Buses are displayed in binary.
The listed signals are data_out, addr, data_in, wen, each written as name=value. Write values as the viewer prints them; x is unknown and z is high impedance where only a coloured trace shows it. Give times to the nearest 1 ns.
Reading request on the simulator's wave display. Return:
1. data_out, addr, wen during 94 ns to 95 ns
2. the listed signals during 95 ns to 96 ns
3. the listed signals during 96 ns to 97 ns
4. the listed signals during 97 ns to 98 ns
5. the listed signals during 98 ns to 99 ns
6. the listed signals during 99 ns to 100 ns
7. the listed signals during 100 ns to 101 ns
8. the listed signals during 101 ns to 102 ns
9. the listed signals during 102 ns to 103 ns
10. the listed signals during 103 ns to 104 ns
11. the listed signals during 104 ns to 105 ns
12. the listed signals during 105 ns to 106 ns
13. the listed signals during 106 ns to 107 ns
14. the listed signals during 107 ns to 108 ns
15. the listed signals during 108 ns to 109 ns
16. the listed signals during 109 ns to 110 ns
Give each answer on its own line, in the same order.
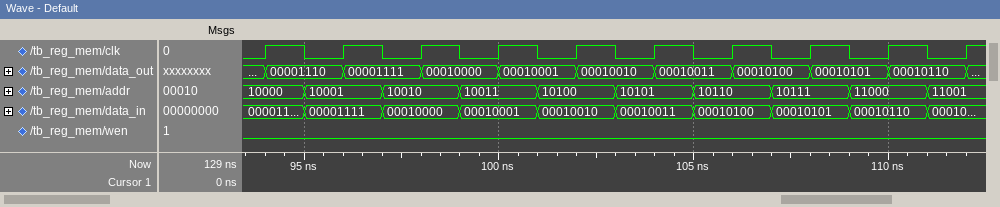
data_out=00001110, addr=10000, wen=0
data_out=00001110, addr=10001, data_in=00001111, wen=0
data_out=00001111, addr=10001, data_in=00001111, wen=0
data_out=00001111, addr=10010, data_in=00010000, wen=0
data_out=00010000, addr=10010, data_in=00010000, wen=0
data_out=00010000, addr=10011, data_in=00010001, wen=0
data_out=00010001, addr=10011, data_in=00010001, wen=0
data_out=00010001, addr=10100, data_in=00010010, wen=0
data_out=00010010, addr=10100, data_in=00010010, wen=0
data_out=00010010, addr=10101, data_in=00010011, wen=0
data_out=00010011, addr=10101, data_in=00010011, wen=0
data_out=00010011, addr=10110, data_in=00010100, wen=0
data_out=00010100, addr=10110, data_in=00010100, wen=0
data_out=00010100, addr=10111, data_in=00010101, wen=0
data_out=00010101, addr=10111, data_in=00010101, wen=0
data_out=00010101, addr=11000, data_in=00010110, wen=0
